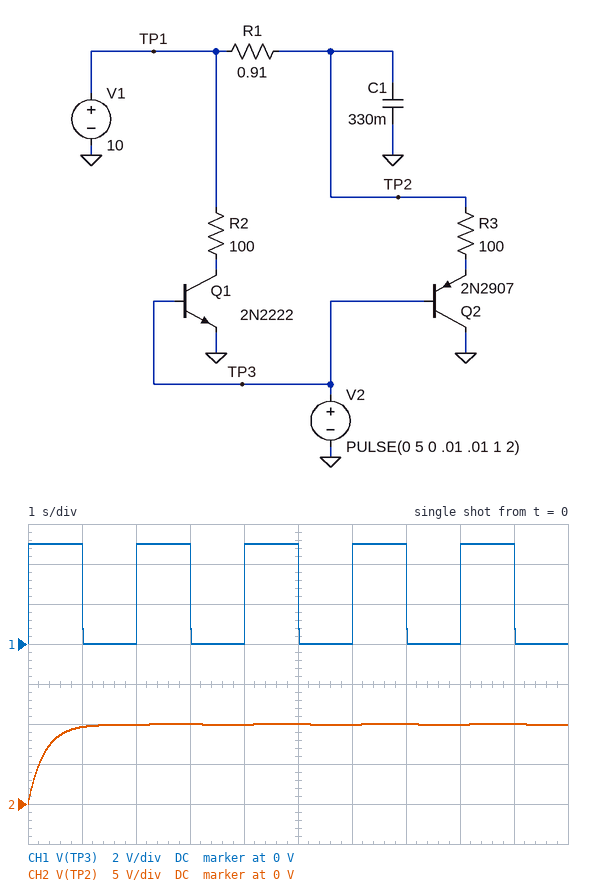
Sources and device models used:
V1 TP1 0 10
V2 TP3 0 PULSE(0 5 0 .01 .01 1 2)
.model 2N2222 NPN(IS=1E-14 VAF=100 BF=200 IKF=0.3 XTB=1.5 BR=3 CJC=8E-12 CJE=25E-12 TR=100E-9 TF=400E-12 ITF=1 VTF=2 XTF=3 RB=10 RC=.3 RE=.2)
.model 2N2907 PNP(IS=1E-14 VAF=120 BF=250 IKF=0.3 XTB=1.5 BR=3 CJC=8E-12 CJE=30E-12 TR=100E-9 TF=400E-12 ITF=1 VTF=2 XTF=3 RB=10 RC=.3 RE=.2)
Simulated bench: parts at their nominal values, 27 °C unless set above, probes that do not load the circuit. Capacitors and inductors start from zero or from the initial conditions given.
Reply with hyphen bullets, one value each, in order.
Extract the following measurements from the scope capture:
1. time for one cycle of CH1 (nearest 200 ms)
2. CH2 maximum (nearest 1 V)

- 2.0 s
- 10 V
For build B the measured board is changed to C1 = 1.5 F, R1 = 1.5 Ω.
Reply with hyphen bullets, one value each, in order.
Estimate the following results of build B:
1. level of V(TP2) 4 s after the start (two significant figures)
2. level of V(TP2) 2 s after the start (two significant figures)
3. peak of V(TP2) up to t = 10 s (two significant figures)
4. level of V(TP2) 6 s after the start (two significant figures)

- 8.3 V
- 5.9 V
- 9.8 V
- 9.2 V
